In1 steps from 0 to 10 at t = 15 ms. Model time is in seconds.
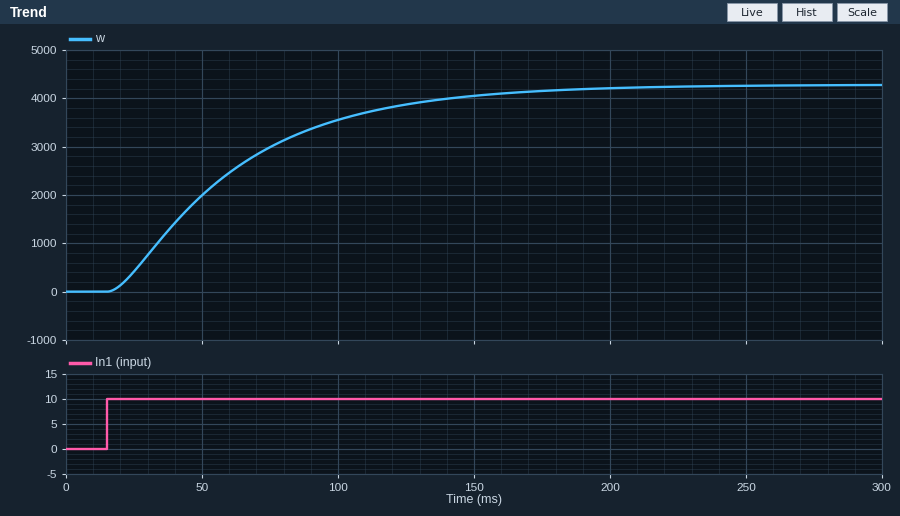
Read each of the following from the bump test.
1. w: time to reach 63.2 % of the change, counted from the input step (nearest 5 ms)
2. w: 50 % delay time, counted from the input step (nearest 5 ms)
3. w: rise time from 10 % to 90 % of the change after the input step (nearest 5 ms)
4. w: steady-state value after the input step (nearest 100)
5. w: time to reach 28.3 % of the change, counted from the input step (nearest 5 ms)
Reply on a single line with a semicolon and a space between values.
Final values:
50 ms; 40 ms; 100 ms; 4300; 20 ms
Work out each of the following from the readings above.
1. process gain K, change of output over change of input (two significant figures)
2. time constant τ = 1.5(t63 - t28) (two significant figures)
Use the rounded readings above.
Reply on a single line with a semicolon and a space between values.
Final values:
430; 45 ms
